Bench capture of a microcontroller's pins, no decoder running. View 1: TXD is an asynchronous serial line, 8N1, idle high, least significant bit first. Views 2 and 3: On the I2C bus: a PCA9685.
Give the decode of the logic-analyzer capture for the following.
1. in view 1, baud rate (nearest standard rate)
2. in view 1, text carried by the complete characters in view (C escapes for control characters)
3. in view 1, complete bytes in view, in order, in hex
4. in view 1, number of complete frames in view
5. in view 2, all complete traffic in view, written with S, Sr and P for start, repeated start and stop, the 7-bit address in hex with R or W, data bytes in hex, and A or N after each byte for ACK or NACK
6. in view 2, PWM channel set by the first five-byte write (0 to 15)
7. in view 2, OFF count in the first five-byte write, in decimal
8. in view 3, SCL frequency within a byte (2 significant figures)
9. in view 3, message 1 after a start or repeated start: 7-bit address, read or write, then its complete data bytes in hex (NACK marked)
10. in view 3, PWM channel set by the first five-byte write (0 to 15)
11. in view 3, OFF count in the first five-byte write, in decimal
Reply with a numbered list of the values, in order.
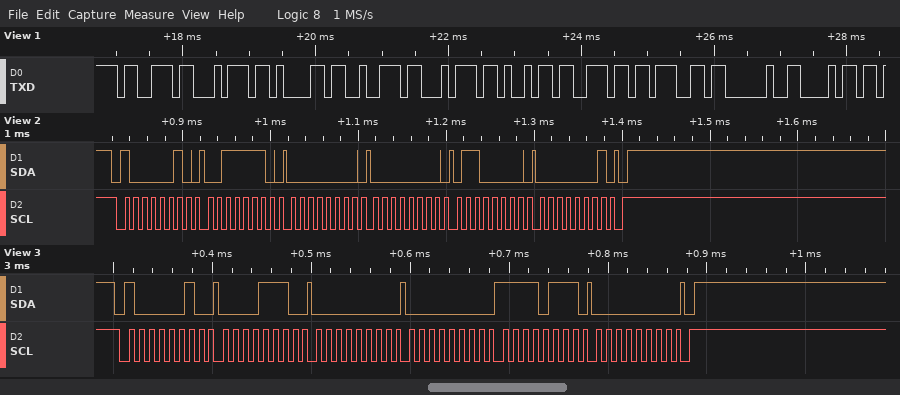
1. 9600 baud
2. "starting h"
3. 73 74 61 72 74 69 6E 67 20 68
4. 10
5. S 41W A 3E A 00 A 00 A 60 A 01 A P
6. 14
7. 352
8. 100 kHz
9. 0x41 write: 0E 00 00 F7 00
10. 2
11. 247
